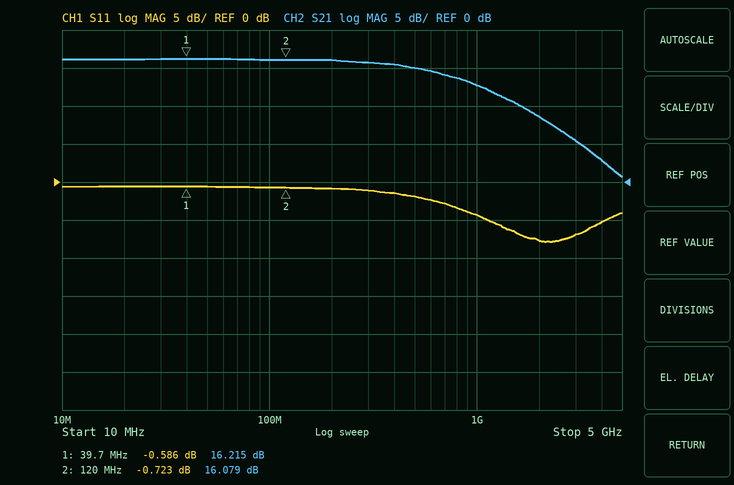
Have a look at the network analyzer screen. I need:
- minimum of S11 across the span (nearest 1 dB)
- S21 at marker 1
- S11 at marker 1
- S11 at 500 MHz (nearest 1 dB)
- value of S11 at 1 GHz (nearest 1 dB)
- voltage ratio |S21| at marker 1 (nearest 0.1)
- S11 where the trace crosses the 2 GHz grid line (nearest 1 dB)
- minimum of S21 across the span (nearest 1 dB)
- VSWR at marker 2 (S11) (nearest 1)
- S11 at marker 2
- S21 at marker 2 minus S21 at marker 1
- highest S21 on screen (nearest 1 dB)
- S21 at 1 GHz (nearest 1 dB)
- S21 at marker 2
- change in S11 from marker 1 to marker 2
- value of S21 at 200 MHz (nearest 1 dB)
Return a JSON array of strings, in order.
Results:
["-8 dB", "16.215 dB", "-0.586 dB", "-2 dB", "-4 dB", "6.5", "-8 dB", "1 dB", "24", "-0.723 dB", "-0.136 dB", "16 dB", "13 dB", "16.079 dB", "-0.137 dB", "16 dB"]
